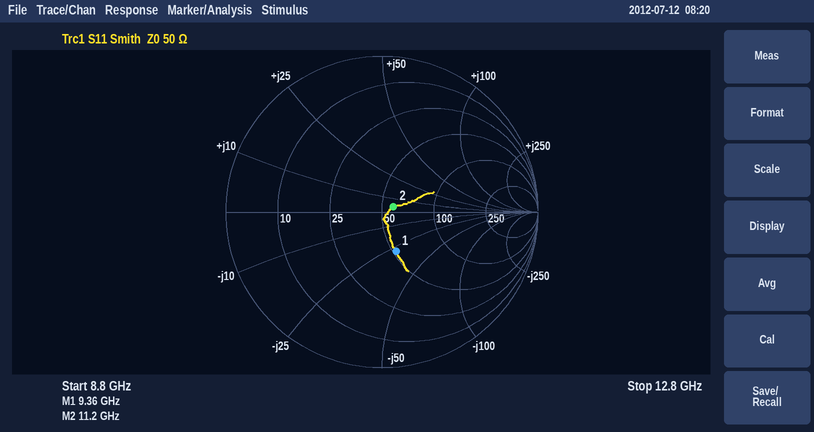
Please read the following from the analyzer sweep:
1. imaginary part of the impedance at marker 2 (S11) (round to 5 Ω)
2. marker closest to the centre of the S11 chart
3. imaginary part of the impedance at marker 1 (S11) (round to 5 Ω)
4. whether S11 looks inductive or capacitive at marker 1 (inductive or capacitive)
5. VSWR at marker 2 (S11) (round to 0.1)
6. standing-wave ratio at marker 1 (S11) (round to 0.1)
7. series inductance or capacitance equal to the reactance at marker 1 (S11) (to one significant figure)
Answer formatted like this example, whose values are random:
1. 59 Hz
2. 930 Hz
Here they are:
1. +5 Ω
2. marker 2
3. -30 Ω
4. capacitive
5. 1.2
6. 1.7
7. 600 fF
